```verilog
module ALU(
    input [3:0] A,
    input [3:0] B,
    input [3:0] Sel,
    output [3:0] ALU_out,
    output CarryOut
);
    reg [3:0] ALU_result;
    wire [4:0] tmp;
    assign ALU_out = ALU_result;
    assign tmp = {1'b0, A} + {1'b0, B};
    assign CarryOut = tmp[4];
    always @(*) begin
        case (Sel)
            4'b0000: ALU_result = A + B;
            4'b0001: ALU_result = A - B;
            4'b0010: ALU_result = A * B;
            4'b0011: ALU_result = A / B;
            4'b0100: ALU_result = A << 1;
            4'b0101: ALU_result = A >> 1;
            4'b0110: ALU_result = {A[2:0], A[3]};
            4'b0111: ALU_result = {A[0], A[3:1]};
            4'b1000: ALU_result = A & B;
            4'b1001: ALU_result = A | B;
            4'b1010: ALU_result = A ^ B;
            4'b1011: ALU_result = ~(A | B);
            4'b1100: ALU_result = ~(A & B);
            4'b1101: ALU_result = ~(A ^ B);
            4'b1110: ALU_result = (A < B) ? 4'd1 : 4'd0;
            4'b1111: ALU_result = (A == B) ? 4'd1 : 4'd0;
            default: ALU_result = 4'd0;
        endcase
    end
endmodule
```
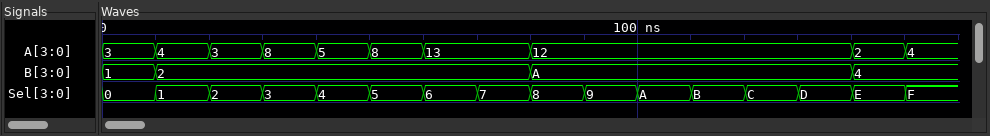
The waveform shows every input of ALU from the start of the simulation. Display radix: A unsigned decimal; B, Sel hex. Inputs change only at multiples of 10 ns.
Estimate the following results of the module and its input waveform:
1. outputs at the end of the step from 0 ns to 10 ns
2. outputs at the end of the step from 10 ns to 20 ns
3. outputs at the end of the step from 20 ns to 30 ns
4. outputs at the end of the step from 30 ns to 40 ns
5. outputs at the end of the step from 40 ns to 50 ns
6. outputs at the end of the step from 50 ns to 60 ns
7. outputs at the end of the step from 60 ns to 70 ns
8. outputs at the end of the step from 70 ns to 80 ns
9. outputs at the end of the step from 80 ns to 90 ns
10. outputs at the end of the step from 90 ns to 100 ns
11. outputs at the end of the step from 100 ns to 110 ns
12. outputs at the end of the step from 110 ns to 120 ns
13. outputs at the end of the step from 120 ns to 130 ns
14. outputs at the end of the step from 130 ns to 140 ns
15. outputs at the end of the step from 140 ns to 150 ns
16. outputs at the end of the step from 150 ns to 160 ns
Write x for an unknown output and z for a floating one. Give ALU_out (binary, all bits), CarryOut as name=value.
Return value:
ALU_out=0100, CarryOut=0
ALU_out=0010, CarryOut=0
ALU_out=0110, CarryOut=0
ALU_out=0100, CarryOut=0
ALU_out=1010, CarryOut=0
ALU_out=0100, CarryOut=0
ALU_out=1011, CarryOut=0
ALU_out=1110, CarryOut=0
ALU_out=1000, CarryOut=1
ALU_out=1110, CarryOut=1
ALU_out=0110, CarryOut=1
ALU_out=0001, CarryOut=1
ALU_out=0111, CarryOut=1
ALU_out=1001, CarryOut=1
ALU_out=0001, CarryOut=0
ALU_out=0001, CarryOut=0
